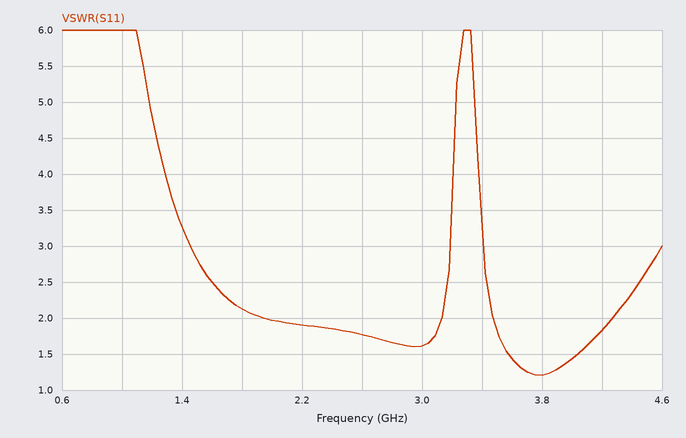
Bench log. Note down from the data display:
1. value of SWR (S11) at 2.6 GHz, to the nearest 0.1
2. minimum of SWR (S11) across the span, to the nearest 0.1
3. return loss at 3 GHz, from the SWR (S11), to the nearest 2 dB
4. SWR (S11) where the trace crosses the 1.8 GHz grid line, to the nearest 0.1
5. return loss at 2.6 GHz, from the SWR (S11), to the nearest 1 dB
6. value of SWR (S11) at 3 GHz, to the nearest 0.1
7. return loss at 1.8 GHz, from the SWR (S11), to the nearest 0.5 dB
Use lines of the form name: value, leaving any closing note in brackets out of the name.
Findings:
value of SWR (S11) at 2.6 GHz, to the nearest 0.1: 1.8
minimum of SWR (S11) across the span, to the nearest 0.1: 1.2
return loss at 3 GHz, from the SWR (S11), to the nearest 2 dB: 12 dB
SWR (S11) where the trace crosses the 1.8 GHz grid line, to the nearest 0.1: 2.1
return loss at 2.6 GHz, from the SWR (S11), to the nearest 1 dB: 11 dB
value of SWR (S11) at 3 GHz, to the nearest 0.1: 1.6
return loss at 1.8 GHz, from the SWR (S11), to the nearest 0.5 dB: 9.0 dB
